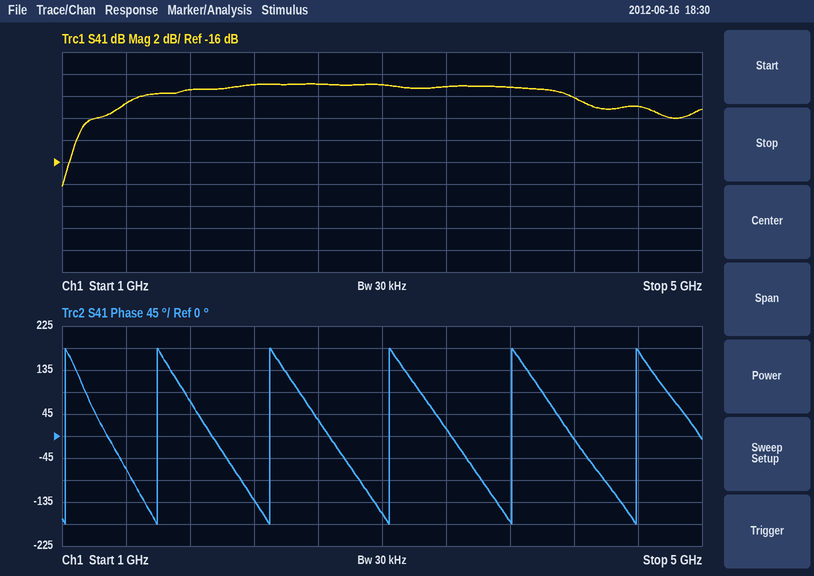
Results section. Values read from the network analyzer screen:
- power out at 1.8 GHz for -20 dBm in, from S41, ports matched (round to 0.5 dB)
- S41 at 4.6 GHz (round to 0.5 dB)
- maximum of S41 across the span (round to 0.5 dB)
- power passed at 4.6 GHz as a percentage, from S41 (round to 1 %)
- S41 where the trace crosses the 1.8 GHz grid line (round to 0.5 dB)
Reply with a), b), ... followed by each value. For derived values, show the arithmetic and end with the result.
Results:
a) -20 dBm + (-9.5 dB) = -29.5 dBm
b) -11.0 dB
c) -9.0 dB
d) 10^(-11/10) ≈ 8 %
e) -9.5 dB
